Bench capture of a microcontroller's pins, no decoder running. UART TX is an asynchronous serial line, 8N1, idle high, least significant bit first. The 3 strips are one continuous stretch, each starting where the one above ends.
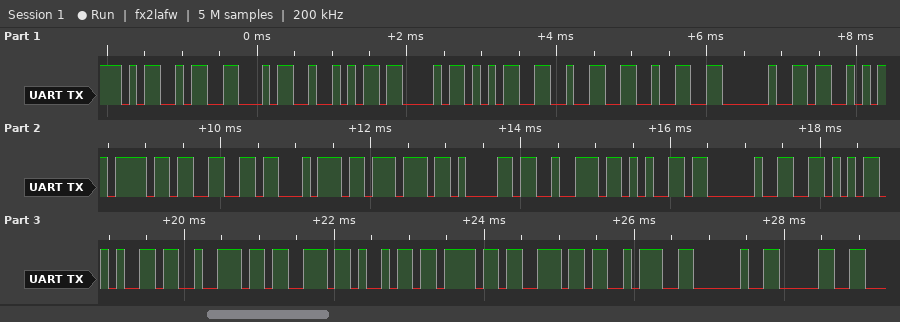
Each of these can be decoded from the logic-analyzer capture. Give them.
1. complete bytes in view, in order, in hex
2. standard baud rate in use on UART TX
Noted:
4D 46 52 43 35 32 32 20 53 6F 66 74 77 61 72 65 20 56 65 72 73 69 6F 6E 3A 20 30
9600 baud
